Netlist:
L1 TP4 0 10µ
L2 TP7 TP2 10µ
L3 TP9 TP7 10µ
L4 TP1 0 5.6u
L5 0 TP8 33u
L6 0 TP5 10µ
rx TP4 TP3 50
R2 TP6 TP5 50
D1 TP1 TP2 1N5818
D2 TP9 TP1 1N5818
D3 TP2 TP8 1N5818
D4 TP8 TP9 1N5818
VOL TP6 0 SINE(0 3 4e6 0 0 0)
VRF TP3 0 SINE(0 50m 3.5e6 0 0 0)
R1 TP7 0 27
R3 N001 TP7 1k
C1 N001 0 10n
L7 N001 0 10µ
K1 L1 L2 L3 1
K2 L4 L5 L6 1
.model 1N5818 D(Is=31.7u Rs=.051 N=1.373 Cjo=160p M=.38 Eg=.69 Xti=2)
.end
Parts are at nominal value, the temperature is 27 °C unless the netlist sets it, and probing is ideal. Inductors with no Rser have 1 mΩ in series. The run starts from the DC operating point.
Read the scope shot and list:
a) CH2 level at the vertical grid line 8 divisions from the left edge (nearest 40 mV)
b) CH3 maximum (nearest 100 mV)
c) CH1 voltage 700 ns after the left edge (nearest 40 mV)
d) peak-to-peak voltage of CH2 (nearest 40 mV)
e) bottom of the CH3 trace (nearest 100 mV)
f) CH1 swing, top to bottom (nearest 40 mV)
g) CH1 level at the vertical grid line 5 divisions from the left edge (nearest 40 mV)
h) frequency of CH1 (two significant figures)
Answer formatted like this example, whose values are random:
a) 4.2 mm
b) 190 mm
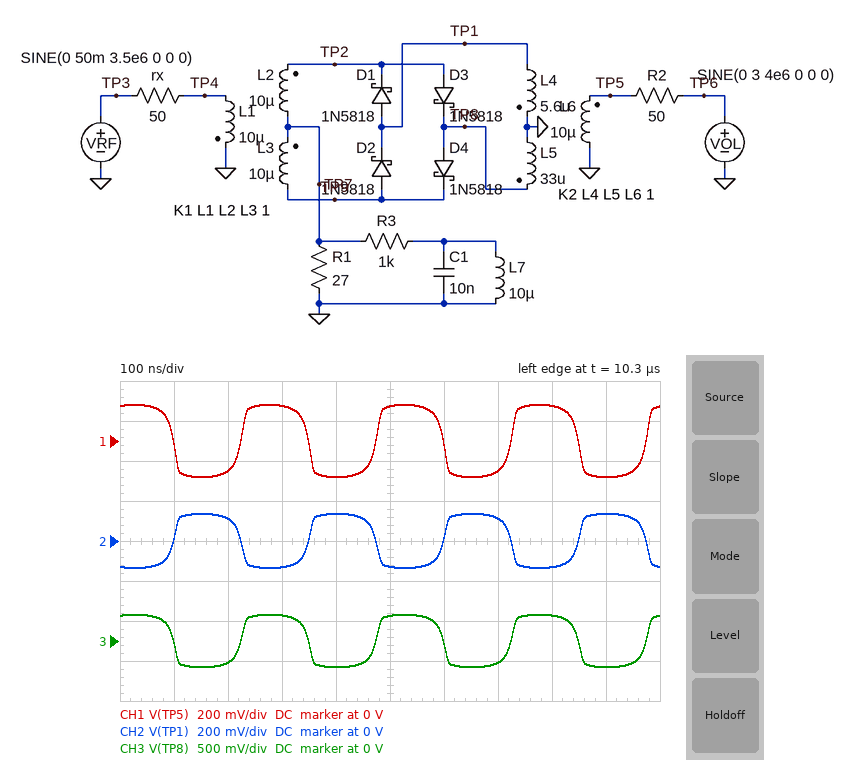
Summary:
a) -120 mV
b) 300 mV
c) -160 mV
d) 280 mV
e) -300 mV
f) 360 mV
g) 160 mV
h) 4.0 MHz
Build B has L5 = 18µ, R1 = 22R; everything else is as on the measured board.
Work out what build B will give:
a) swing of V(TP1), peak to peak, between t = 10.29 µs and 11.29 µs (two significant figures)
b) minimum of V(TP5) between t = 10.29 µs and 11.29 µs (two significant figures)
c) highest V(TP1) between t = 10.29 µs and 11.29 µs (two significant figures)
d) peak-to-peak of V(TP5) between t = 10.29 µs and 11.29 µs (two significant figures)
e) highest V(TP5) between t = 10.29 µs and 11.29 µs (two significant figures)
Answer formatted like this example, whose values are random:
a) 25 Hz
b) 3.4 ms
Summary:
a) 340 mV
b) -230 mV
c) 170 mV
d) 460 mV
e) 230 mV
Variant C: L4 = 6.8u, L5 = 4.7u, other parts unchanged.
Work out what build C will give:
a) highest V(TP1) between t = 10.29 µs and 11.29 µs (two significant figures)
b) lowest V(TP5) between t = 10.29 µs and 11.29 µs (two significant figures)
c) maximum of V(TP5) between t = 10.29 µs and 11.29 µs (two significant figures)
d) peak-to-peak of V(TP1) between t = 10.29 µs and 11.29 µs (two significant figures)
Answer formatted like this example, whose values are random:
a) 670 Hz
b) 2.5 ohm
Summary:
a) 270 mV
b) -330 mV
c) 330 mV
d) 550 mV
